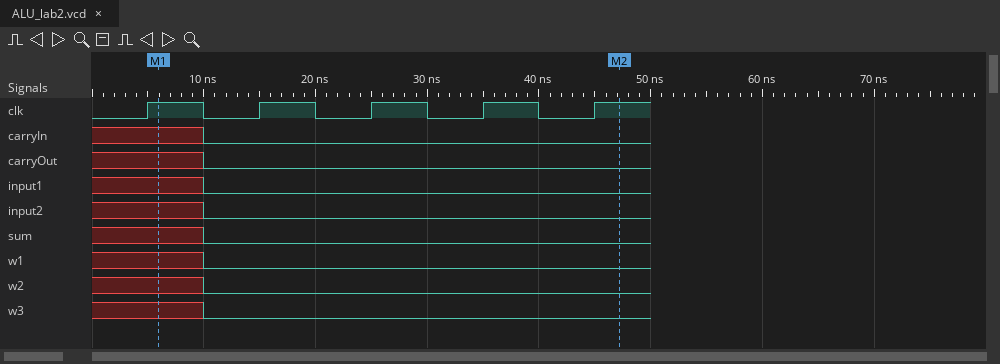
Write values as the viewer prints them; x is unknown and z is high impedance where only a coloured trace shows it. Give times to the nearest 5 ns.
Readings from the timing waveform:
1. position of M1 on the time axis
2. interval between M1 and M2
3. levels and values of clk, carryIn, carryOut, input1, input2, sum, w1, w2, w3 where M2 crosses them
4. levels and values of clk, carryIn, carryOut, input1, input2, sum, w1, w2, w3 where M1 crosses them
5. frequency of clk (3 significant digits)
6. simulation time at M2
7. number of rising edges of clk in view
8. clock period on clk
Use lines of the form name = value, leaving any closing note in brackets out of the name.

position of M1 on the time axis = 5 ns
interval between M1 and M2 = 40 ns
levels and values of clk, carryIn, carryOut, input1, input2, sum, w1, w2, w3 where M2 crosses them = clk=1, carryIn=0, carryOut=0, input1=0, input2=0, sum=0, w1=0, w2=0, w3=0
levels and values of clk, carryIn, carryOut, input1, input2, sum, w1, w2, w3 where M1 crosses them = clk=1, carryIn=x, carryOut=x, input1=x, input2=x, sum=x, w1=x, w2=x, w3=x
frequency of clk = 100 MHz
simulation time at M2 = 45 ns
number of rising edges of clk in view = 5
clock period on clk = 10 ns
